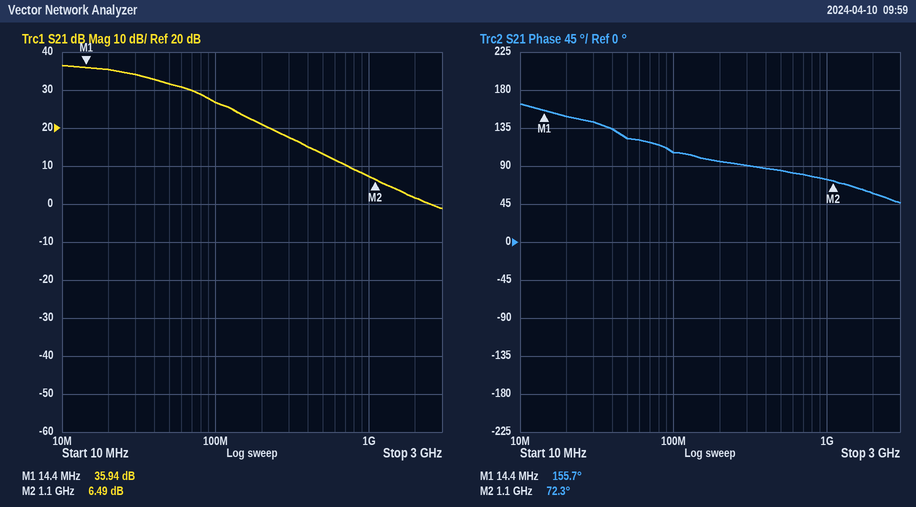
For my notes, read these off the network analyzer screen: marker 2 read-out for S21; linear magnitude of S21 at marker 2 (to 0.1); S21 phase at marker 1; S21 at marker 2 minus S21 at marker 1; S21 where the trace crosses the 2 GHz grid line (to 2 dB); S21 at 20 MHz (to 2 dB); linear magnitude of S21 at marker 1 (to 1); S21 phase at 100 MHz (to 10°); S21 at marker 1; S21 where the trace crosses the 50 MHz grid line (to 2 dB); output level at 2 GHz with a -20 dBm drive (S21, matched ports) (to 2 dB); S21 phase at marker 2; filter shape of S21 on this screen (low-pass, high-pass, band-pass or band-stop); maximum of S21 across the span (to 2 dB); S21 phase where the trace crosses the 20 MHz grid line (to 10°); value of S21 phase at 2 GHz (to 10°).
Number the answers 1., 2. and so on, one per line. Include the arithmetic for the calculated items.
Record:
1. 6.49 dB
2. 10^(6.49/20) ≈ 2.1
3. 155.7°
4. 6.49 − (35.94) = -29.45 dB
5. 2 dB
6. 36 dB
7. 10^(35.94/20) ≈ 63
8. 110°
9. 35.94 dB
10. 32 dB
11. -20 dBm + (2 dB) = -18 dBm
12. 72.3°
13. low-pass
14. 36 dB
15. 150°
16. 60°
